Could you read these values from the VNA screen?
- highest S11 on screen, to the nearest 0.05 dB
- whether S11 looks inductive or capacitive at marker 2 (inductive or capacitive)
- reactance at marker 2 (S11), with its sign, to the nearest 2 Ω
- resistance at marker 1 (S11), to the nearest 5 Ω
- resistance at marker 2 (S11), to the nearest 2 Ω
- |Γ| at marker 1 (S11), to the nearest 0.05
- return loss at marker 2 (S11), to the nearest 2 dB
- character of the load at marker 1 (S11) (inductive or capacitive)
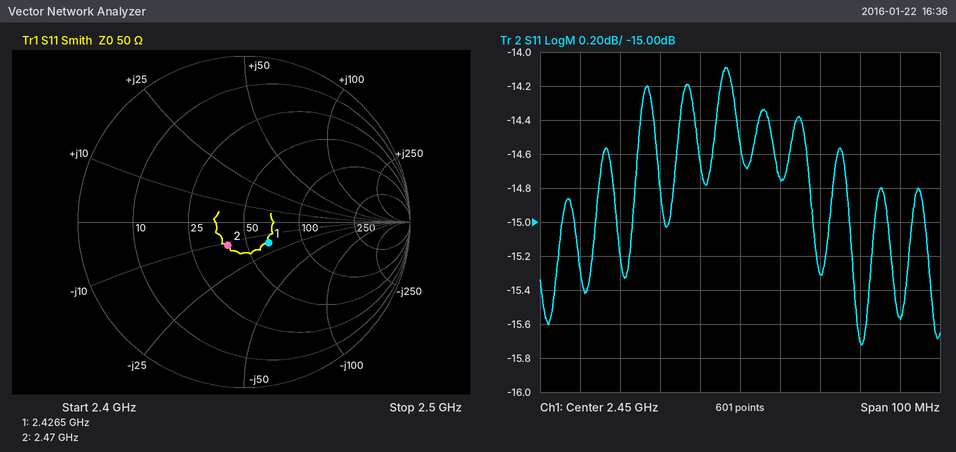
-14.10 dB
capacitive
-12 Ω
65 Ω
40 Ω
0.20
16 dB
capacitive
